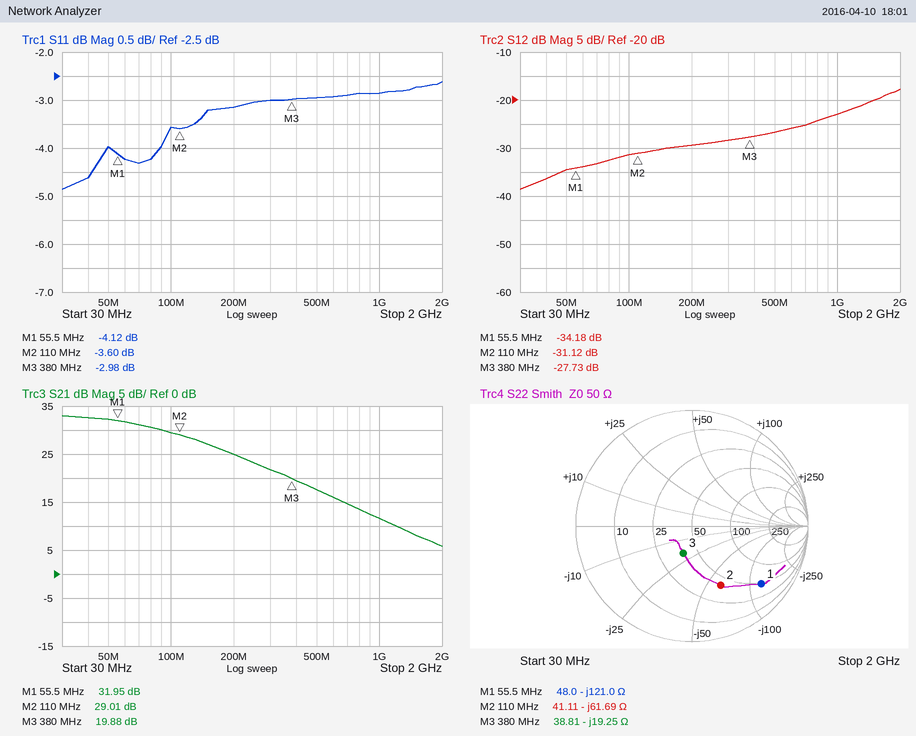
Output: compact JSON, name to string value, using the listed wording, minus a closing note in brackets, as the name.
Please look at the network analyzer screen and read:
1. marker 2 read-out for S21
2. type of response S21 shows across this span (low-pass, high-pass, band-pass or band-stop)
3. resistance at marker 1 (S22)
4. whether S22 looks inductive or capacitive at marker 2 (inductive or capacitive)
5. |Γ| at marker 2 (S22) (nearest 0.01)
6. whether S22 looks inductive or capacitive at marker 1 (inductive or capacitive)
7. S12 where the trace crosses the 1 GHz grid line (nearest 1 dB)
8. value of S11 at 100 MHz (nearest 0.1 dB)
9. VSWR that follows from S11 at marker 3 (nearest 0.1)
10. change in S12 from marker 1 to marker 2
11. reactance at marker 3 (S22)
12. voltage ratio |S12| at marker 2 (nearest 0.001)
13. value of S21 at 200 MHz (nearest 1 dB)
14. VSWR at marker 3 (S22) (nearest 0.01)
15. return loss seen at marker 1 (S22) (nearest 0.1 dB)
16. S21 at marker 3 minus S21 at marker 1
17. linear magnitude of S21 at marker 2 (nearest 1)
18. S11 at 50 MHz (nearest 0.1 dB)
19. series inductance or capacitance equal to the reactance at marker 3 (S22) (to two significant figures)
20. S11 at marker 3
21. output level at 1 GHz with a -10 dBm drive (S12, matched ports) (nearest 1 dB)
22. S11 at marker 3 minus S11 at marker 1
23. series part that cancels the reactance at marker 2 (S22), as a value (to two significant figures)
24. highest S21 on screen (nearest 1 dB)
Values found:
{"marker 2 read-out for S21": "29.01 dB", "type of response S21 shows across this span": "low-pass", "resistance at marker 1": "48.0 Ω", "whether S22 looks inductive or capacitive at marker 2": "capacitive", "|Γ| at marker 2 (S22)": "0.57", "whether S22 looks inductive or capacitive at marker 1": "capacitive", "S12 where the trace crosses the 1 GHz grid line": "-23 dB", "value of S11 at 100 MHz": "-3.6 dB", "VSWR that follows from S11 at marker 3": "5.9", "change in S12 from marker 1 to marker 2": "3.06 dB", "reactance at marker 3": "-19.25 Ω", "voltage ratio |S12| at marker 2": "0.028", "value of S21 at 200 MHz": "25 dB", "VSWR at marker 3 (S22)": "1.65", "return loss seen at marker 1 (S22)": "2.2 dB", "S21 at marker 3 minus S21 at marker 1": "-12.07 dB", "linear magnitude of S21 at marker 2": "28", "S11 at 50 MHz": "-4.0 dB", "series inductance or capacitance equal to the reactance at marker 3 (S22)": "22 pF", "S11 at marker 3": "-2.98 dB", "output level at 1 GHz with a -10 dBm drive (S12, matched ports)": "-33 dBm", "S11 at marker 3 minus S11 at marker 1": "1.14 dB", "series part that cancels the reactance at marker 2 (S22), as a value": "89 nH", "highest S21 on screen": "33 dB"}
